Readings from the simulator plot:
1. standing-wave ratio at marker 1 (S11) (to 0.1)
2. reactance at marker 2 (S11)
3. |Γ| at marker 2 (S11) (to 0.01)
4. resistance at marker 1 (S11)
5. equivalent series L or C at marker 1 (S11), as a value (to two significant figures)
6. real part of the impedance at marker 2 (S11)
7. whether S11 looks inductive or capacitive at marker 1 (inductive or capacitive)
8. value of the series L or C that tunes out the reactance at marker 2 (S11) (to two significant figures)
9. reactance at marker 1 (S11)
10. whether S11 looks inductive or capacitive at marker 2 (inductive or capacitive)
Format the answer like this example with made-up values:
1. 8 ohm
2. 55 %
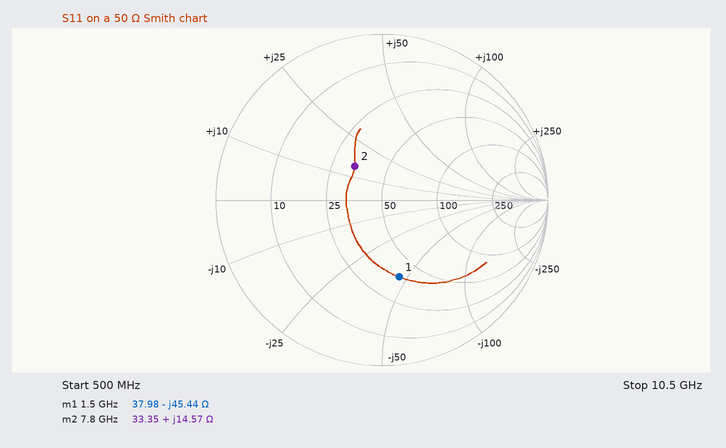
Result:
1. 2.8
2. +14.57 Ω
3. 0.26
4. 37.98 Ω
5. 2.3 pF
6. 33.35 Ω
7. capacitive
8. 1.4 pF
9. -45.44 Ω
10. inductive
